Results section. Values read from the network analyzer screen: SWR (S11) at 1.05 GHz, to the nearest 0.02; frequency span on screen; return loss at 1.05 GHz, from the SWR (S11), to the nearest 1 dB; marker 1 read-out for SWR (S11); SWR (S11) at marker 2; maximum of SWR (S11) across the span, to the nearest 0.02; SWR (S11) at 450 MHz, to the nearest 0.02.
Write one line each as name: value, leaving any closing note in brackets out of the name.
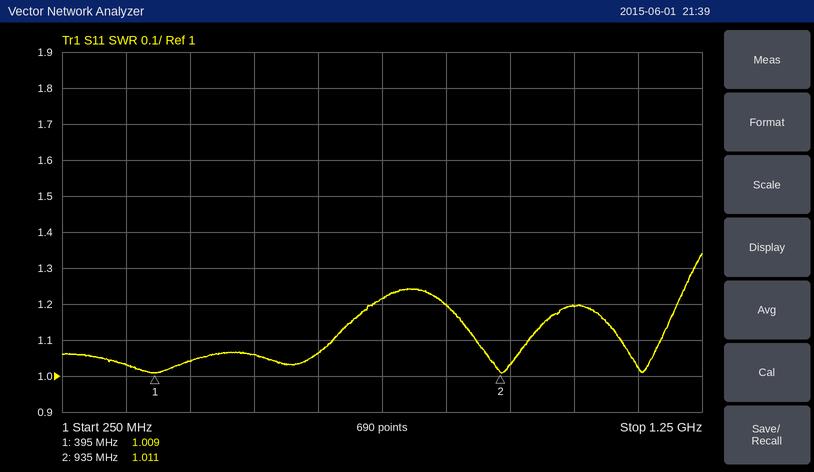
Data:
SWR (S11) at 1.05 GHz, to the nearest 0.02: 1.20
frequency span on screen: 1 GHz
return loss at 1.05 GHz, from the SWR (S11), to the nearest 1 dB: 21 dB
marker 1 read-out for SWR: 1.009
SWR (S11) at marker 2: 1.011
maximum of SWR (S11) across the span, to the nearest 0.02: 1.34
SWR (S11) at 450 MHz, to the nearest 0.02: 1.04
